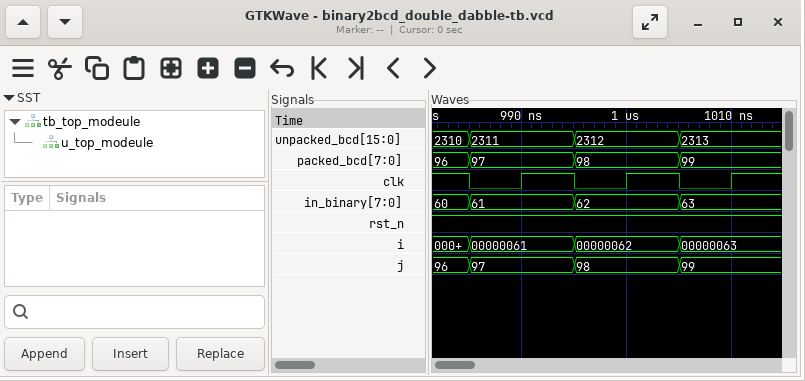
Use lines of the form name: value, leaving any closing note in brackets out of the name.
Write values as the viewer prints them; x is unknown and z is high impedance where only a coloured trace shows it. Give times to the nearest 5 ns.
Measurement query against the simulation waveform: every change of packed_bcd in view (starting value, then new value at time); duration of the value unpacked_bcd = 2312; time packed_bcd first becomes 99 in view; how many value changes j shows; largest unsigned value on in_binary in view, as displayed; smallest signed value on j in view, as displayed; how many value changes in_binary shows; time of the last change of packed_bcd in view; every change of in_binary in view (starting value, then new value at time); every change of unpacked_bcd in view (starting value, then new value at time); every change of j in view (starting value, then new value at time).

every change of packed_bcd in view: 96, 97 at 985 ns, 98 at 995 ns, 99 at 1005 ns
duration of the value unpacked_bcd = 2312: 10 ns
time packed_bcd first becomes 99 in view: 1005 ns
how many value changes j shows: 3
largest unsigned value on in_binary in view, as displayed: 63
smallest signed value on j in view, as displayed: 96
how many value changes in_binary shows: 3
time of the last change of packed_bcd in view: 1005 ns
every change of in_binary in view: 60, 61 at 985 ns, 62 at 995 ns, 63 at 1005 ns
every change of unpacked_bcd in view: 2310, 2311 at 985 ns, 2312 at 995 ns, 2313 at 1005 ns
every change of j in view: 96, 97 at 985 ns, 98 at 995 ns, 99 at 1005 ns
